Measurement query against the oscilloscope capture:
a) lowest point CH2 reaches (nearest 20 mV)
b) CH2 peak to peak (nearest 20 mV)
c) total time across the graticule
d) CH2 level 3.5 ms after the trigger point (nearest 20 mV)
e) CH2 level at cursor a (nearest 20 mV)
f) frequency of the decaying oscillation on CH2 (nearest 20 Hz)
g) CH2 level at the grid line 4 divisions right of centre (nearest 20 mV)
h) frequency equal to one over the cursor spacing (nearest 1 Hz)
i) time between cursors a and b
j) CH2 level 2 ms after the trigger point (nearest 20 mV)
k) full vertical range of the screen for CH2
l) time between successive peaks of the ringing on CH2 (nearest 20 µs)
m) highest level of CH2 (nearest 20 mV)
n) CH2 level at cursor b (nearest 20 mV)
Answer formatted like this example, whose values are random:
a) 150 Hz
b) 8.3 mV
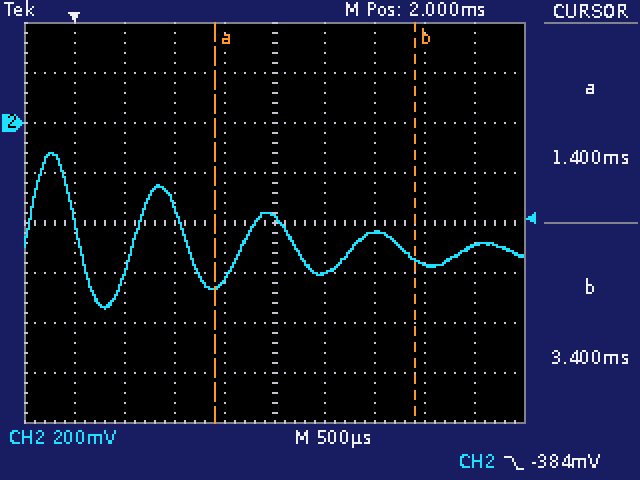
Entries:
a) -740 mV
b) 620 mV
c) 5 ms
d) -560 mV
e) -660 mV
f) 920 Hz
g) -480 mV
h) 500 Hz
i) 2.00 ms
j) -380 mV
k) 1.6 V
l) 1.08 ms
m) -120 mV
n) -540 mV
